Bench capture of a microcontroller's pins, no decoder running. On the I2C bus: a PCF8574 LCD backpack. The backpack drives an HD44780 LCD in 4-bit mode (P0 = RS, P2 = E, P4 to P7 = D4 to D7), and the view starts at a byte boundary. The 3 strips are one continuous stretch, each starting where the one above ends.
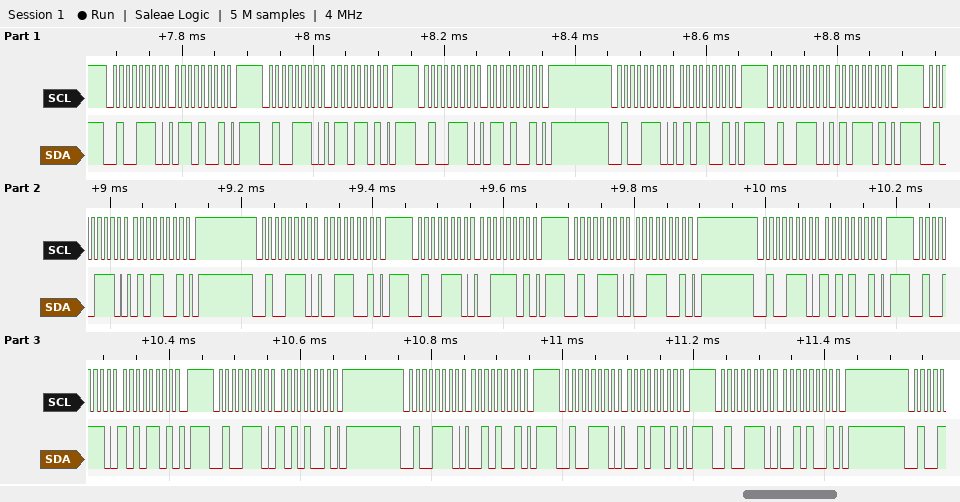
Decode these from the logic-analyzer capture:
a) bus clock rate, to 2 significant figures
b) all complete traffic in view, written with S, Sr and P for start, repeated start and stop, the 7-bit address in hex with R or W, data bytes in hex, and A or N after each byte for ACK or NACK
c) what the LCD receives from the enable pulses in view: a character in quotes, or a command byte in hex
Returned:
100 kHz
S 27W A 69 A P S 27W A 6D A P S 27W A 69 A P S 27W A 59 A P S 27W A 5D A P S 27W A 59 A P S 27W A 39 A P S 27W A 3D A P S 27W A 39 A P S 27W A A9 A P S 27W A AD A P S 27W A A9 A P S 27W A 29 A P S 27W A 2D A P S 27W A 29 A P
'e' ':'
